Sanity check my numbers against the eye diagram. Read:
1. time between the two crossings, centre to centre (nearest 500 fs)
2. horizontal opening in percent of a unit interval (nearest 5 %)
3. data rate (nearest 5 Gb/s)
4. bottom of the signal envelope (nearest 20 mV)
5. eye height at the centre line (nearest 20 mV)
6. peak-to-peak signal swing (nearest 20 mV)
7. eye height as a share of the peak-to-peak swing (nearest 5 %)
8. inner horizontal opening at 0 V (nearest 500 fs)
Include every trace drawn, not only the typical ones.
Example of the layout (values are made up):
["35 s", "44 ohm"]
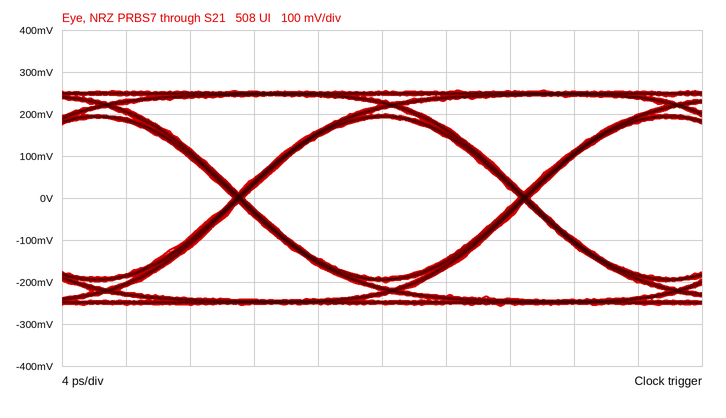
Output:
["18.0 ps", "95 %", "55 Gb/s", "-260 mV", "380 mV", "520 mV", "75 %", "17.0 ps"]
